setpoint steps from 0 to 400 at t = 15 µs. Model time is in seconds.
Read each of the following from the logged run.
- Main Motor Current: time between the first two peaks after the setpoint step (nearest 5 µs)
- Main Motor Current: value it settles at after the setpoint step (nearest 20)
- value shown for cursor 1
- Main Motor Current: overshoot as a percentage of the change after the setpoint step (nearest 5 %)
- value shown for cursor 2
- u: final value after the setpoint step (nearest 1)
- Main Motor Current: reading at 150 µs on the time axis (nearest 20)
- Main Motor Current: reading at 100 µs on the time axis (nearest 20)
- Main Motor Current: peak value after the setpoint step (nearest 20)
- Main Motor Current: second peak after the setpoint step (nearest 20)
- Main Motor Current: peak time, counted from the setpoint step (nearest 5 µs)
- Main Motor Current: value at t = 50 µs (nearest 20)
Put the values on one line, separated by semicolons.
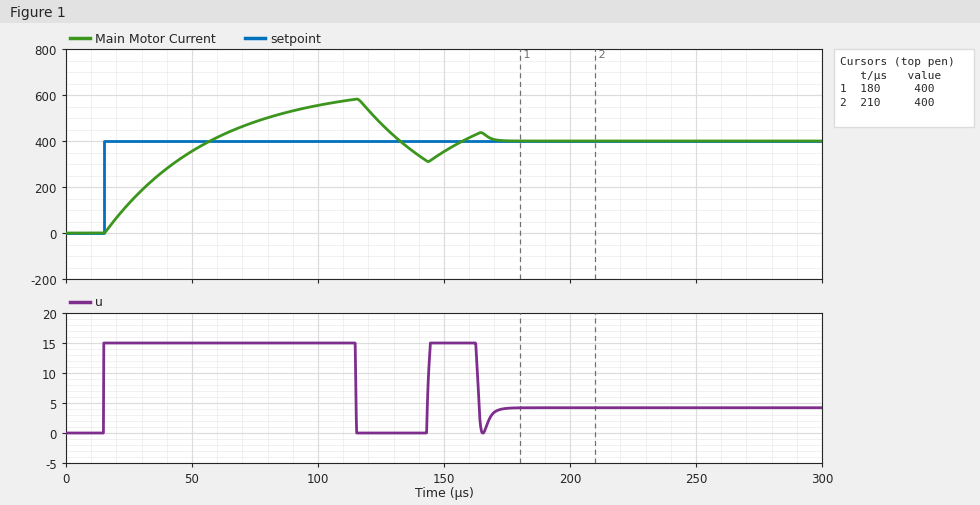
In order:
50 µs; 400; 400; 45 %; 400; 4; 360; 560; 580; 440; 100 µs; 360
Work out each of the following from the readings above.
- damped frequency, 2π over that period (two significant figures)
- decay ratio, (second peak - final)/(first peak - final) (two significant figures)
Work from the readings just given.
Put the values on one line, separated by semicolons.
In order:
0.13 rad/µs; 0.22
